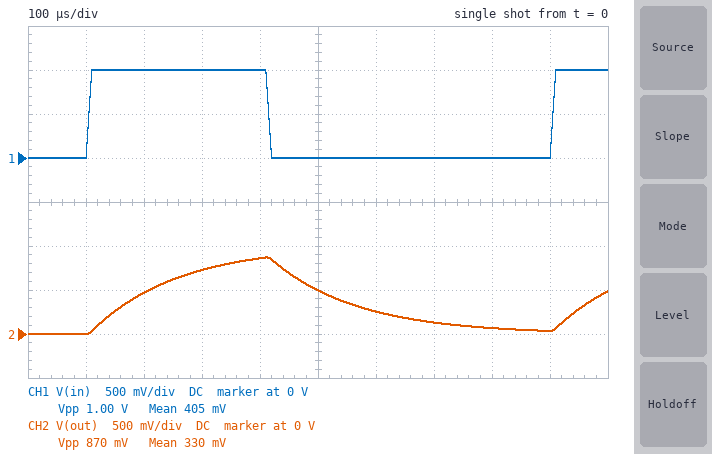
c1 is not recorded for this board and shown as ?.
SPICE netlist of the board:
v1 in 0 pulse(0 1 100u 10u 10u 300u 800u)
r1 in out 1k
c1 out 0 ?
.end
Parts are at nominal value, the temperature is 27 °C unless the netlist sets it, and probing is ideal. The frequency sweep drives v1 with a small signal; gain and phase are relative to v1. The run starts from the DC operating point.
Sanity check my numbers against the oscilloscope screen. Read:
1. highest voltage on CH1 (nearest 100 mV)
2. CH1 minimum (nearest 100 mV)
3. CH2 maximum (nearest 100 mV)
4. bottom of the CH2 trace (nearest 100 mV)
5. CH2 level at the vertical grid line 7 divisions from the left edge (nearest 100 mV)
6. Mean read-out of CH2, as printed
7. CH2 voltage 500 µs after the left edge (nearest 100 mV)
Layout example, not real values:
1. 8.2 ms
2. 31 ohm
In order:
1. 1.0 V
2. 0 V
3. 900 mV
4. 0 V
5. 100 mV
6. 330 mV
7. 500 mV
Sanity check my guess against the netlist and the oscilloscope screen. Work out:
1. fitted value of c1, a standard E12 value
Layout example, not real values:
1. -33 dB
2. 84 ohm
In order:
1. 150 nF
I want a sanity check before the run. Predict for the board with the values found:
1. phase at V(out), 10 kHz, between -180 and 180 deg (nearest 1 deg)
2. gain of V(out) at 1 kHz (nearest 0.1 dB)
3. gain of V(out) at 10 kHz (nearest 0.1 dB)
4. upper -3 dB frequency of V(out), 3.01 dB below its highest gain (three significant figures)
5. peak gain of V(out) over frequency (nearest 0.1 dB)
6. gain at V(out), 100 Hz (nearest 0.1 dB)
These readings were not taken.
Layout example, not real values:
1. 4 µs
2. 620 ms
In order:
1. -84 deg
2. -2.8 dB
3. -19.5 dB
4. 1.06 kHz
5. 0 dB
6. 0 dB
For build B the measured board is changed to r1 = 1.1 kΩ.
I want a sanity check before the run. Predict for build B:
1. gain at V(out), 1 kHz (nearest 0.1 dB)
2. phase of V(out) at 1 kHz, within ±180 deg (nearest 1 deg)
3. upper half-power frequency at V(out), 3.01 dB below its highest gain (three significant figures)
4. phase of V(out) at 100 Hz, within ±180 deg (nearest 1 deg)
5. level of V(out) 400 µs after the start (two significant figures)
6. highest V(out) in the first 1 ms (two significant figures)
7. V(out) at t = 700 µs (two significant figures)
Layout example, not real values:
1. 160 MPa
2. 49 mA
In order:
1. -3.2 dB
2. -46 deg
3. 965 Hz
4. -6 deg
5. 830 mV
6. 840 mV
7. 150 mV
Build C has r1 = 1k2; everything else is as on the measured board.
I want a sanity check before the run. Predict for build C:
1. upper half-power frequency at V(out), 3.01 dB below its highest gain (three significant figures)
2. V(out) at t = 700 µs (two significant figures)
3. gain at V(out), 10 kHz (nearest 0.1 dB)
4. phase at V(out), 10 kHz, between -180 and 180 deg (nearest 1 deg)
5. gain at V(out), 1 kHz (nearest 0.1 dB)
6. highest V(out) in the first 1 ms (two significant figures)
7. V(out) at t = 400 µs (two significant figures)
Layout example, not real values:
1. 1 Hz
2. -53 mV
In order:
1. 884 Hz
2. 170 mV
3. -21.1 dB
4. -85 deg
5. -3.6 dB
6. 820 mV
7. 810 mV
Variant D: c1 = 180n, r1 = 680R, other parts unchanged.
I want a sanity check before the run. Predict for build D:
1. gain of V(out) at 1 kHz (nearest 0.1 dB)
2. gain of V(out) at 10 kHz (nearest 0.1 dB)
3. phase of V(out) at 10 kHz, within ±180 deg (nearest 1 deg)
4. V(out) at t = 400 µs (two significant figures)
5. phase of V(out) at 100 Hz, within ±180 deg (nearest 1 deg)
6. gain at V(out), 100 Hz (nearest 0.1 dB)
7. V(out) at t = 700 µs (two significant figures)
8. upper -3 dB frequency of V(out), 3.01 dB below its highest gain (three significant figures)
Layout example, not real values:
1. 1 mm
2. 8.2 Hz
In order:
1. -2.0 dB
2. -17.8 dB
3. -83 deg
4. 910 mV
5. -4 deg
6. 0 dB
7. 90 mV
8. 1.30 kHz
